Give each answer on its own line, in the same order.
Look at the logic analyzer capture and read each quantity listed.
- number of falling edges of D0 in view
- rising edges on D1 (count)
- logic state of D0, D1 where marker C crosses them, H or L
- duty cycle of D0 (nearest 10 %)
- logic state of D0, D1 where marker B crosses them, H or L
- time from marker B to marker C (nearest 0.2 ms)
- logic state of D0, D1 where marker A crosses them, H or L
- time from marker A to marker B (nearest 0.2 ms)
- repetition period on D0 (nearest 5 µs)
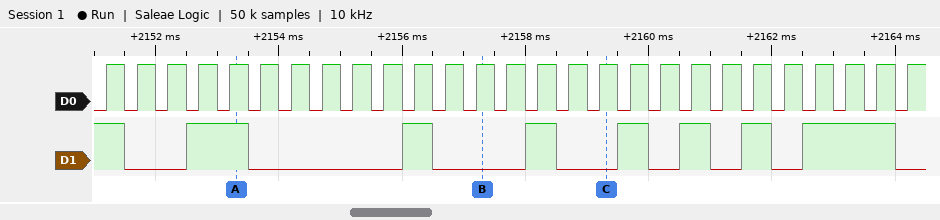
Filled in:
26
7
D0=H, D1=L
60 %
D0=H, D1=L
2 ms
D0=H, D1=H
4 ms
500 µs
